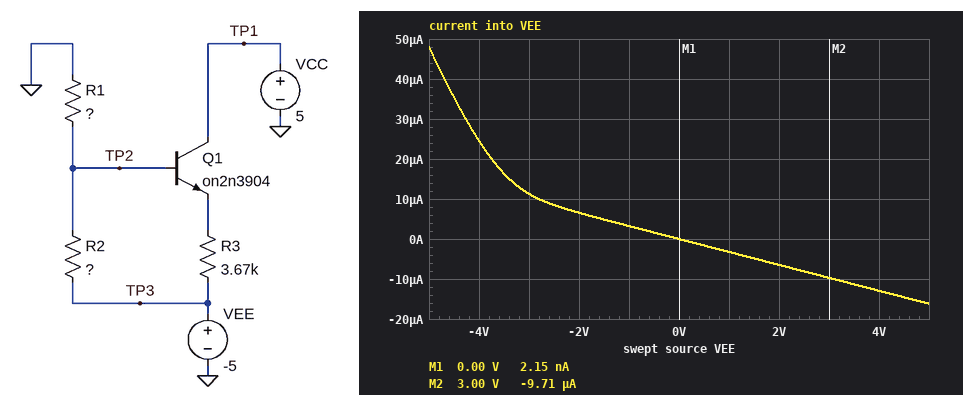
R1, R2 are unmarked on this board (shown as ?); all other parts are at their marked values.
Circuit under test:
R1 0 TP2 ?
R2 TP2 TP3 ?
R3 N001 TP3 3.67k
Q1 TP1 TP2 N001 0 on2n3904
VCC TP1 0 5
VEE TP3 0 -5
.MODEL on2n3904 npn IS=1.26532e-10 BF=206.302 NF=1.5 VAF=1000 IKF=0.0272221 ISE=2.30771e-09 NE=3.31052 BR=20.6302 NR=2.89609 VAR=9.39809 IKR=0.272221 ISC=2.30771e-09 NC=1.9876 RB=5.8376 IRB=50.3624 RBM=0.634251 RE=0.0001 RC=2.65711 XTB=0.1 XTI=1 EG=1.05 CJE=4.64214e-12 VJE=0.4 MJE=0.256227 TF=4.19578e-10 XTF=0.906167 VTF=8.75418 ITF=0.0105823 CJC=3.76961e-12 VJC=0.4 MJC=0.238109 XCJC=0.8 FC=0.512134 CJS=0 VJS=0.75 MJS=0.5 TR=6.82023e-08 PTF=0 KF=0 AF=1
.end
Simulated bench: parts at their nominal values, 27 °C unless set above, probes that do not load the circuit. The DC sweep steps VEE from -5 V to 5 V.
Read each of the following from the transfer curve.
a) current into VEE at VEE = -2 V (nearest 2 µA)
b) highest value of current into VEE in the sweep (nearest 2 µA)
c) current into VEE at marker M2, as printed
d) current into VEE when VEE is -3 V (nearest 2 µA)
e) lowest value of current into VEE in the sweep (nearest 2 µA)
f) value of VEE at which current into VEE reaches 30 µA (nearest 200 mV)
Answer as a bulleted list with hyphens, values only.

- 6 µA
- 48 µA
- -9.71 µA
- 12 µA
- -16 µA
- -4.2 V
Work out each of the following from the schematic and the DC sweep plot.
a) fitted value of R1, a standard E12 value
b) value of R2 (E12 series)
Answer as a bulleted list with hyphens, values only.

- 270 kΩ
- 39 kΩ
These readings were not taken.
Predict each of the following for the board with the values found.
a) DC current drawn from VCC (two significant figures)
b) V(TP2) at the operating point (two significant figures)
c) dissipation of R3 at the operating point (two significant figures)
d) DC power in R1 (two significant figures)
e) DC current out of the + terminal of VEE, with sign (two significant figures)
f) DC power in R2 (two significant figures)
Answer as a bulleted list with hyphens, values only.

- 32 µA
- -4.4 V
- 3.9 µW
- 72 µW
- -48 µA
- 9.3 µW
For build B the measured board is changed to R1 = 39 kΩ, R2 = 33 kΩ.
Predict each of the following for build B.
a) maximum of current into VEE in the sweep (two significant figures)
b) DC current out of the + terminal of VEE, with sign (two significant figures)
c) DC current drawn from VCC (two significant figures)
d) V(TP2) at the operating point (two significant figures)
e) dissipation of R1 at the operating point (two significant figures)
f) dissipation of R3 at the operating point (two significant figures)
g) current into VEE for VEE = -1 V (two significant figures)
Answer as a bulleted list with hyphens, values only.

- 510 µA
- -510 µA
- 440 µA
- -2.8 V
- 200 µW
- 720 µW
- 21 µA
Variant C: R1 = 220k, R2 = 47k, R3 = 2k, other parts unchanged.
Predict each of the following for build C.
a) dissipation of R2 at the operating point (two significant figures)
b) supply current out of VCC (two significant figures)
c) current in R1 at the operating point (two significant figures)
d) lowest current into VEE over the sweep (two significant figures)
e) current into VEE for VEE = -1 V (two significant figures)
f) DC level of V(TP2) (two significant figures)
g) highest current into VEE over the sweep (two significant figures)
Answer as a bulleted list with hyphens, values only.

- 14 µW
- 130 µA
- 19 µA
- -19 µA
- 3.8 µA
- -4.2 V
- 150 µA
